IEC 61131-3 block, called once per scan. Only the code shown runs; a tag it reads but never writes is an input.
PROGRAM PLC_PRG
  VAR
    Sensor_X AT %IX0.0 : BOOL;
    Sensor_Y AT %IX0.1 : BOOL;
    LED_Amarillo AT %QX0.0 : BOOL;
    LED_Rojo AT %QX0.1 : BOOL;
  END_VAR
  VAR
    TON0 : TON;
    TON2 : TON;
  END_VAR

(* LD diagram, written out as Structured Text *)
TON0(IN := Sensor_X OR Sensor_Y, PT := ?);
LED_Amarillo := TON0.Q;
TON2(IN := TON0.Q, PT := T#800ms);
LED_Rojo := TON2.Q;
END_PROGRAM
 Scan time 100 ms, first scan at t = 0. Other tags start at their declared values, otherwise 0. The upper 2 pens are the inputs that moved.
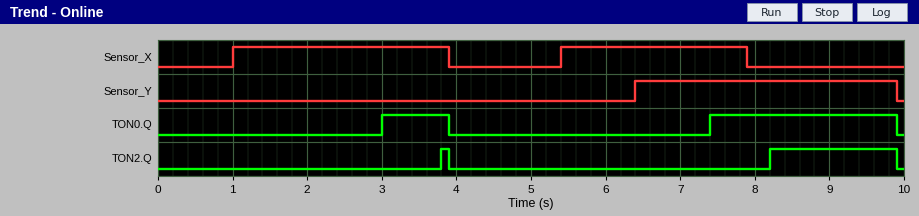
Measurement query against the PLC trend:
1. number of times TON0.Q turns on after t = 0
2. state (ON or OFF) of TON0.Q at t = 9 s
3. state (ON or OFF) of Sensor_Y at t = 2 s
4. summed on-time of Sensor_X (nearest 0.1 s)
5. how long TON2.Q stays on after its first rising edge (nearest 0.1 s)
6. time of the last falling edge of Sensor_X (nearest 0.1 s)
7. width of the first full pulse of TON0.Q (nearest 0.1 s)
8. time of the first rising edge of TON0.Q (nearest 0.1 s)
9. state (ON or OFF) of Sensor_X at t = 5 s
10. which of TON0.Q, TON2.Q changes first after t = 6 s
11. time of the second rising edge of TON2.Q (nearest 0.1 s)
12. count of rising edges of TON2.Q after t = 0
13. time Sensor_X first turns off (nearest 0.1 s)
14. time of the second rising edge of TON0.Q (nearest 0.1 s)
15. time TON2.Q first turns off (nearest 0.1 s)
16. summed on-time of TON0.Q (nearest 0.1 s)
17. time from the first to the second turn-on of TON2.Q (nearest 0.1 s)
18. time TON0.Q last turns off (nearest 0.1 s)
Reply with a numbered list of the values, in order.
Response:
1. 2
2. ON
3. OFF
4. 5.4 s
5. 0.1 s
6. 7.9 s
7. 0.9 s
8. 3.0 s
9. OFF
10. TON0.Q
11. 8.2 s
12. 2
13. 3.9 s
14. 7.4 s
15. 3.9 s
16. 3.4 s
17. 4.4 s
18. 9.9 s
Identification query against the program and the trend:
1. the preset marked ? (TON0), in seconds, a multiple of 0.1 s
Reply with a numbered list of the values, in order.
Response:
1. 2.0 s
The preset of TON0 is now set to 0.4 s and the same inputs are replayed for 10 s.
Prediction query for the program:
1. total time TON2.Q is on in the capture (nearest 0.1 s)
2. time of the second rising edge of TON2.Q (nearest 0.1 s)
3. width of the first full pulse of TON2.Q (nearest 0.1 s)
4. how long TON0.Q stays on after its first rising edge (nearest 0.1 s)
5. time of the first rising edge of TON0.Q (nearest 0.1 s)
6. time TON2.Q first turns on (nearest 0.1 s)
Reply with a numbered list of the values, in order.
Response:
1. 5.0 s
2. 6.6 s
3. 1.7 s
4. 2.5 s
5. 1.4 s
6. 2.2 s
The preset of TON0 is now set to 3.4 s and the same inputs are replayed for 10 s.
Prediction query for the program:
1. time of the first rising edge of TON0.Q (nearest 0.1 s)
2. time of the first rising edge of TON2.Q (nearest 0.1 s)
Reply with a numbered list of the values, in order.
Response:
1. 8.8 s
2. 9.6 s
